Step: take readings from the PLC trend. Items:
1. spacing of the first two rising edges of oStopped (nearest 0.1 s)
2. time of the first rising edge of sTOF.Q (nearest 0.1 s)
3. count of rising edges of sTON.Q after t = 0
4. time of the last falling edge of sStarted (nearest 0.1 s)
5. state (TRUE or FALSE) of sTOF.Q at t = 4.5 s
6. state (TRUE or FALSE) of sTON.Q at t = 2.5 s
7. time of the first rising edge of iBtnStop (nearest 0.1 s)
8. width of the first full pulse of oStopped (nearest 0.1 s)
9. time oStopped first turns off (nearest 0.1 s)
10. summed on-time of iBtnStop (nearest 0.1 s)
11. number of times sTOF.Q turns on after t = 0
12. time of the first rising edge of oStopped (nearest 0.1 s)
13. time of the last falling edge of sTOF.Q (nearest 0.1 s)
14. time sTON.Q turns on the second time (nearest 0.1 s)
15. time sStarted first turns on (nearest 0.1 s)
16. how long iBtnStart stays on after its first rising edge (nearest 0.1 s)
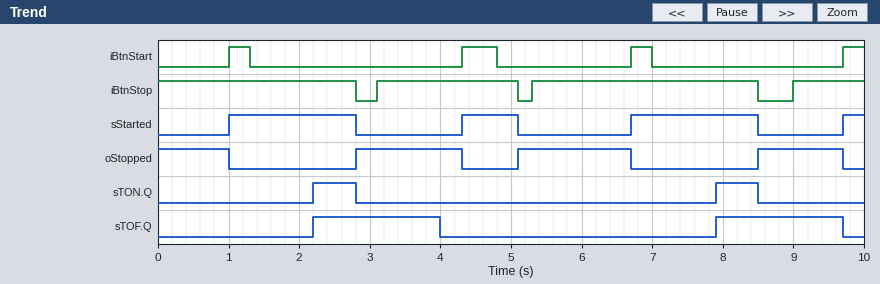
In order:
2.3 s
2.2 s
2
8.5 s
FALSE
TRUE
3.1 s
1.5 s
1.0 s
9.0 s
2
2.8 s
9.7 s
7.9 s
1.0 s
0.3 s
